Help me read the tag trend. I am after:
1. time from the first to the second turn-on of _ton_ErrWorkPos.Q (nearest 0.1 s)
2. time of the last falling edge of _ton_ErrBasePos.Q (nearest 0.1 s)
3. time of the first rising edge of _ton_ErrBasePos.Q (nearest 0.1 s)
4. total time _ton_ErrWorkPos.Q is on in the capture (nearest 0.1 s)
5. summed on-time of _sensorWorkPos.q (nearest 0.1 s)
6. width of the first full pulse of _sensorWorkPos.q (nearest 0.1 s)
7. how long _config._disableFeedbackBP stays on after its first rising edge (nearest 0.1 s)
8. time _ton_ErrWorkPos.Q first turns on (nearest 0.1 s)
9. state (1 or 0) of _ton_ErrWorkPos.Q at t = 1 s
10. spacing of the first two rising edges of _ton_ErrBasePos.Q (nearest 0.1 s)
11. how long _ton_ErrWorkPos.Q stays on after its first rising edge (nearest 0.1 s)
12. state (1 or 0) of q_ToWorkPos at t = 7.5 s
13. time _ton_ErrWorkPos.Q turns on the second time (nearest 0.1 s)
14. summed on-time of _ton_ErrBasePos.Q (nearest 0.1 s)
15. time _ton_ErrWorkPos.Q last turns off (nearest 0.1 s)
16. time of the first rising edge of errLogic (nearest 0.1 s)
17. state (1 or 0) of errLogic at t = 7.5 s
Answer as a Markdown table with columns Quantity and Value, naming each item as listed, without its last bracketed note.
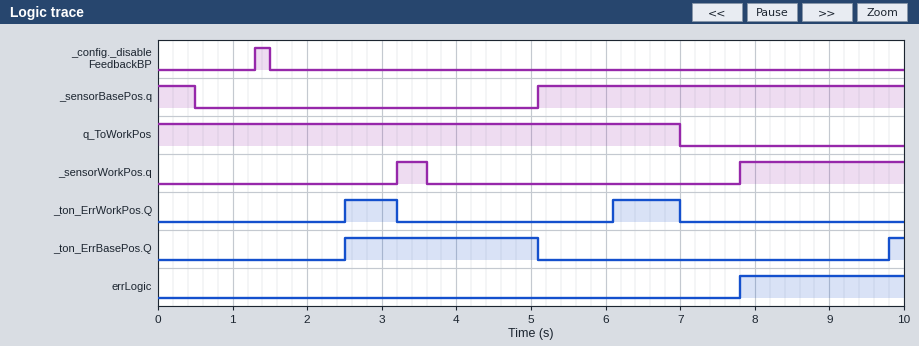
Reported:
| Quantity | Value |
|---|---|
| time from the first to the second turn-on of _ton_ErrWorkPos.Q | 3.6 s |
| time of the last falling edge of _ton_ErrBasePos.Q | 5.1 s |
| time of the first rising edge of _ton_ErrBasePos.Q | 2.5 s |
| total time _ton_ErrWorkPos.Q is on in the capture | 1.6 s |
| summed on-time of _sensorWorkPos.q | 2.6 s |
| width of the first full pulse of _sensorWorkPos.q | 0.4 s |
| how long _config._disableFeedbackBP stays on after its first rising edge | 0.2 s |
| time _ton_ErrWorkPos.Q first turns on | 2.5 s |
| state (1 or 0) of _ton_ErrWorkPos.Q at t = 1 s | 0 |
| spacing of the first two rising edges of _ton_ErrBasePos.Q | 7.3 s |
| how long _ton_ErrWorkPos.Q stays on after its first rising edge | 0.7 s |
| state (1 or 0) of q_ToWorkPos at t = 7.5 s | 0 |
| time _ton_ErrWorkPos.Q turns on the second time | 6.1 s |
| summed on-time of _ton_ErrBasePos.Q | 2.8 s |
| time _ton_ErrWorkPos.Q last turns off | 7.0 s |
| time of the first rising edge of errLogic | 7.8 s |
| state (1 or 0) of errLogic at t = 7.5 s | 0 |
